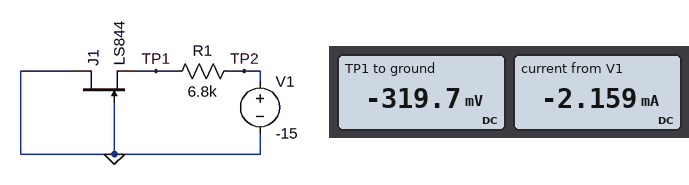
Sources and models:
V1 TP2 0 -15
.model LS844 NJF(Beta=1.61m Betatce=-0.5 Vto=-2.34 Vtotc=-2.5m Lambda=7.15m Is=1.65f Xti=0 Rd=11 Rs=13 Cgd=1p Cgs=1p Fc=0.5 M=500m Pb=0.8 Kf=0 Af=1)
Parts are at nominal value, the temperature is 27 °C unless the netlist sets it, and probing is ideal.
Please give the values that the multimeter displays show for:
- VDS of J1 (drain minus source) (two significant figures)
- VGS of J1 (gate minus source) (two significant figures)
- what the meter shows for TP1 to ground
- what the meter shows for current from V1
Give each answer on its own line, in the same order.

320 mV
320 mV
-319.7 mV
-2.159 mA
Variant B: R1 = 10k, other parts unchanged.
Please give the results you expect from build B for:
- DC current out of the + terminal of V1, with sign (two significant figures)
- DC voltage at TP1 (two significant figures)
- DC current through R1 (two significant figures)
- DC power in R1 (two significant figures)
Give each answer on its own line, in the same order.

-1.5 mA
-220 mV
1.5 mA
22 mW
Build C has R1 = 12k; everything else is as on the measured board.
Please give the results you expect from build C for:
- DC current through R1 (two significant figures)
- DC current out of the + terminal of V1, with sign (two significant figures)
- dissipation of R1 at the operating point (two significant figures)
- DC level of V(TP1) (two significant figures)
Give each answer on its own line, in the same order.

1.2 mA
-1.2 mA
18 mW
-190 mV
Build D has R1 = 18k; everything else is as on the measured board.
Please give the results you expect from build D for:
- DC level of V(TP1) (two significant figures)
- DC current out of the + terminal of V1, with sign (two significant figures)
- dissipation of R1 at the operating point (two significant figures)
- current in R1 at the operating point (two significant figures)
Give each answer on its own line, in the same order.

-130 mV
-830 µA
12 mW
830 µA
